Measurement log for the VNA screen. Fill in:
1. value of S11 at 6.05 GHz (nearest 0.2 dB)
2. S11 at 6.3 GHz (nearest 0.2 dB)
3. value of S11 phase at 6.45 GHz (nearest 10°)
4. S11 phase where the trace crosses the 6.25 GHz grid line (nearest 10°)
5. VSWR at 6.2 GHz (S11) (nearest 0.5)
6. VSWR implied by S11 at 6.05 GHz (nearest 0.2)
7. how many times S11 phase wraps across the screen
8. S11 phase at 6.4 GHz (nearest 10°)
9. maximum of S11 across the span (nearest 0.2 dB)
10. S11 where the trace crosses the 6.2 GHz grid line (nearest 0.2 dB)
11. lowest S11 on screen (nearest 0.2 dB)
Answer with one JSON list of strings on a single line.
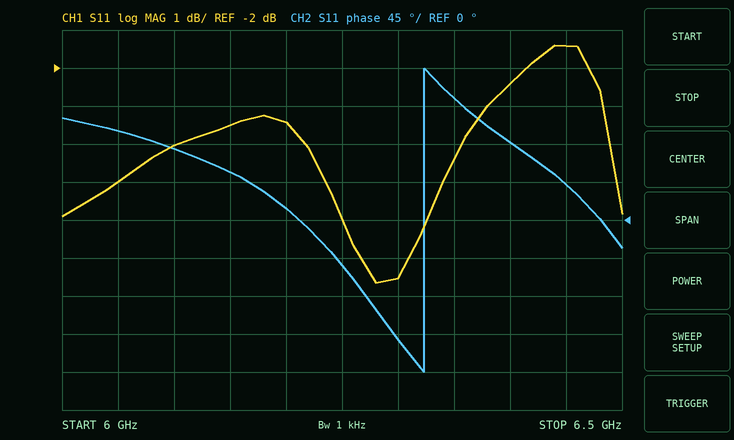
["-5.0 dB", "-7.6 dB", "40°", "-50°", "5.0", "3.6", "1", "90°", "-1.4 dB", "-3.4 dB", "-7.6 dB"]
